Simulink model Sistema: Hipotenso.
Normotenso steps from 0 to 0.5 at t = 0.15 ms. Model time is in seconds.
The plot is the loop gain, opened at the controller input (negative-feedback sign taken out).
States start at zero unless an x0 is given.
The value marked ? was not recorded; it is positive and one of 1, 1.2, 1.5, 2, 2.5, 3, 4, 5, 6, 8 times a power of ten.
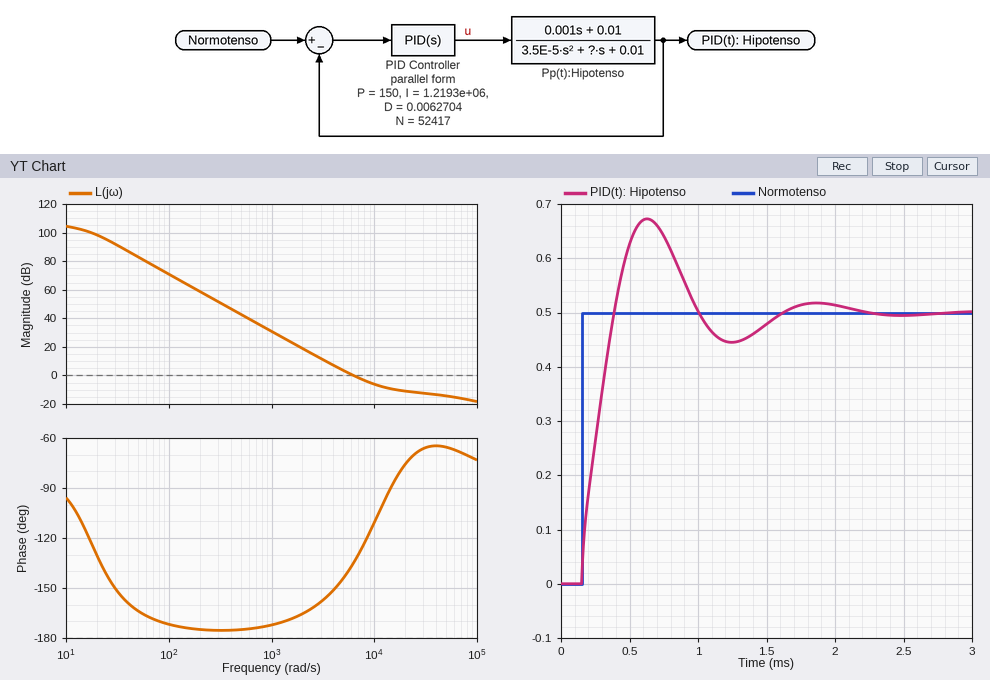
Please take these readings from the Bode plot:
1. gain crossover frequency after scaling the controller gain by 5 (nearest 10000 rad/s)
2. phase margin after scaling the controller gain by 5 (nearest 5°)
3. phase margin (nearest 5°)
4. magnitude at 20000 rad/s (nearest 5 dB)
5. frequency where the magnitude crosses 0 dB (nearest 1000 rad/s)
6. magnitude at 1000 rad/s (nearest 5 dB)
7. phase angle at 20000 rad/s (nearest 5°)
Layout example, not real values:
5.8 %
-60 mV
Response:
50000 rad/s
115°
45°
-10 dB
6000 rad/s
30 dB
-75°
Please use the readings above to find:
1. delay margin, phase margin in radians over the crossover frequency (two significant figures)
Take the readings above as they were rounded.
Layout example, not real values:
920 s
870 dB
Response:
0.00013 s
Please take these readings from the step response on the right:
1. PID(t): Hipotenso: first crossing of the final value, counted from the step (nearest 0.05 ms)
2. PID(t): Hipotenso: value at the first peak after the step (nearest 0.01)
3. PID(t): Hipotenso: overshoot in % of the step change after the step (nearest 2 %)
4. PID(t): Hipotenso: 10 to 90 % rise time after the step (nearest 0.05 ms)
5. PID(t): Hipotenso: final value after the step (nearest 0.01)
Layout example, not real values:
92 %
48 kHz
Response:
0.25 ms
0.67
34 %
0.20 ms
0.50
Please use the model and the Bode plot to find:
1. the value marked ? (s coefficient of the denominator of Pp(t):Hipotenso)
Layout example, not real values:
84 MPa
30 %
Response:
0.0008
